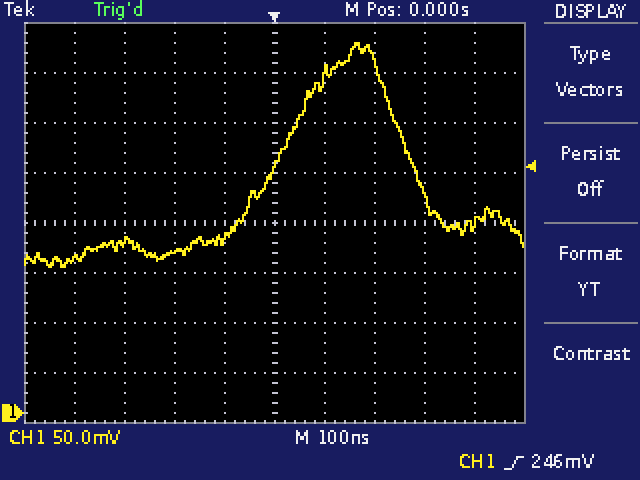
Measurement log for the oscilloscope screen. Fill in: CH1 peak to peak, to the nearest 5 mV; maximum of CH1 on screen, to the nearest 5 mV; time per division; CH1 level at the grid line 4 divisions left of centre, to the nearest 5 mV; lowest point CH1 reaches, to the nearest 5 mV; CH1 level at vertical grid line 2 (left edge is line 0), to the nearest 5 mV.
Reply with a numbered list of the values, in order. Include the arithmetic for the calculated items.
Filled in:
1. 370 mV − (145 mV) = 225 mV
2. 370 mV
3. 100 ns
4. 155 mV
5. 145 mV
6. 170 mV
